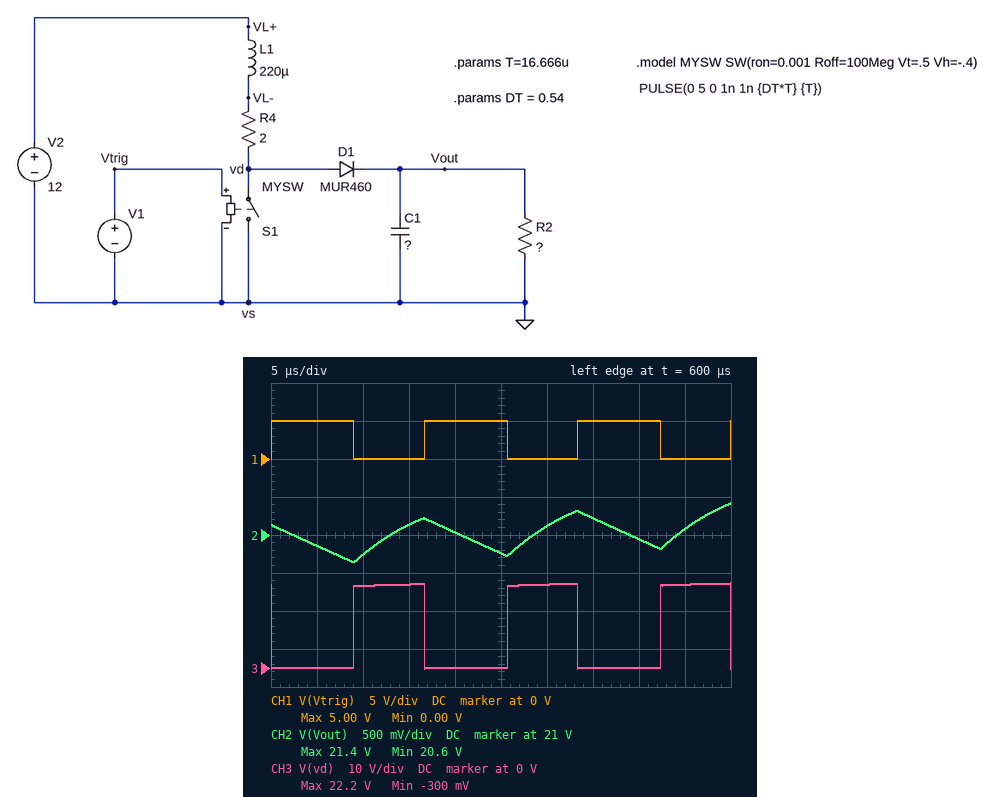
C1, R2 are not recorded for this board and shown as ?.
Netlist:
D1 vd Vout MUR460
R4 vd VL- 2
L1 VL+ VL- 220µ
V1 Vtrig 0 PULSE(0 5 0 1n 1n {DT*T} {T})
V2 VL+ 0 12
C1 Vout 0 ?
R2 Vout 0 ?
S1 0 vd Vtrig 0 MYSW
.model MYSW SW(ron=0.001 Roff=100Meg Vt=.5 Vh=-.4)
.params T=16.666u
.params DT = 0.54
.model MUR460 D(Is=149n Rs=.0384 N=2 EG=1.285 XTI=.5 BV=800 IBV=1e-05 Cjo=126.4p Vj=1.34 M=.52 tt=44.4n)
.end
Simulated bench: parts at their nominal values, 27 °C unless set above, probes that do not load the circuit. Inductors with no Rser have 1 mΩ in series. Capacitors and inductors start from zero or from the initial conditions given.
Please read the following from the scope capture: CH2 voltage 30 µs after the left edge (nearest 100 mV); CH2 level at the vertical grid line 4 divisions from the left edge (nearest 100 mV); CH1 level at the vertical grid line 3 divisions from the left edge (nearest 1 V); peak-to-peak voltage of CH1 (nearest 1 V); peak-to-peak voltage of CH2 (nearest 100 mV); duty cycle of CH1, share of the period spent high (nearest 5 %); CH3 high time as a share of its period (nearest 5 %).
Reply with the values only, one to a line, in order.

21.1 V
21.0 V
0 V
5 V
800 mV
55 %
45 %
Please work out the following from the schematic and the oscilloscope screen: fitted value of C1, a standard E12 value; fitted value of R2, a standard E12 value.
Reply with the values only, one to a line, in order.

6.8 µF
56 Ω
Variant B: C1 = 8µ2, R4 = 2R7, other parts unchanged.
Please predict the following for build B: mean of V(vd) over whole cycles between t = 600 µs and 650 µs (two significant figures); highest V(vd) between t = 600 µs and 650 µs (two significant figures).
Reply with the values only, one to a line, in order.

9.8 V
21 V
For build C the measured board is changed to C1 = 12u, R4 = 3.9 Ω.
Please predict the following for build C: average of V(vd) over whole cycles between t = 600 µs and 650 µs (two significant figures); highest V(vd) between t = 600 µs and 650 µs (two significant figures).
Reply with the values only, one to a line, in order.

9.1 V
20 V
